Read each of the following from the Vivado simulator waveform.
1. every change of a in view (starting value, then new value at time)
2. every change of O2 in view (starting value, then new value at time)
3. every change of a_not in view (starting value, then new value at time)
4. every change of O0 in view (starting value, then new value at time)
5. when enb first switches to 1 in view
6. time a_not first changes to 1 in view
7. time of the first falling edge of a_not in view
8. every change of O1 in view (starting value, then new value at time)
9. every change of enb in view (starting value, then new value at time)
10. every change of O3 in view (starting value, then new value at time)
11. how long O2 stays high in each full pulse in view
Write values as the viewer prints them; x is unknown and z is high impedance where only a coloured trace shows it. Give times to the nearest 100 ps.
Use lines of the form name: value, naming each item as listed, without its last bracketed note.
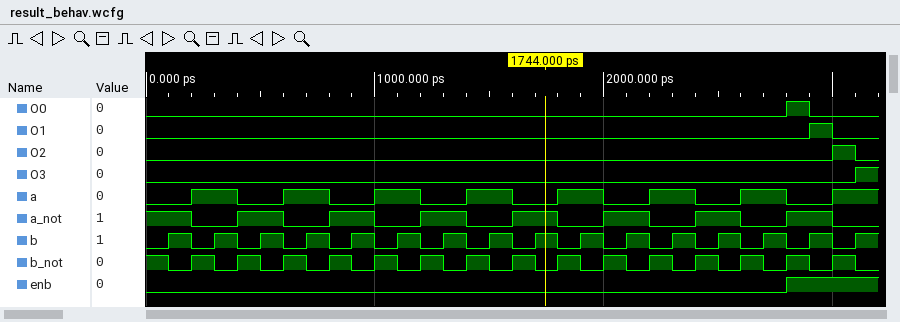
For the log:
every change of a in view: 0, 1 at 200 ps, 0 at 400 ps, 1 at 600 ps, 0 at 800 ps, 1 at 1000 ps, 0 at 1200 ps, 1 at 1400 ps, 0 at 1600 ps, 1 at 1800 ps, 0 at 2000 ps, 1 at 2200 ps, 0 at 2400 ps, 1 at 2600 ps, 0 at 2800 ps, 1 at 3000 ps
every change of O2 in view: 0, 1 at 3000 ps, 0 at 3100 ps
every change of a_not in view: 1, 0 at 200 ps, 1 at 400 ps, 0 at 600 ps, 1 at 800 ps, 0 at 1000 ps, 1 at 1200 ps, 0 at 1400 ps, 1 at 1600 ps, 0 at 1800 ps, 1 at 2000 ps, 0 at 2200 ps, 1 at 2400 ps, 0 at 2600 ps, 1 at 2800 ps, 0 at 3000 ps
every change of O0 in view: 0, 1 at 2800 ps, 0 at 2900 ps
when enb first switches to 1 in view: 2800 ps
time a_not first changes to 1 in view: 400 ps
time of the first falling edge of a_not in view: 200 ps
every change of O1 in view: 0, 1 at 2900 ps, 0 at 3000 ps
every change of enb in view: 0, 1 at 2800 ps
every change of O3 in view: 0, 1 at 3100 ps
how long O2 stays high in each full pulse in view: 100 ps
